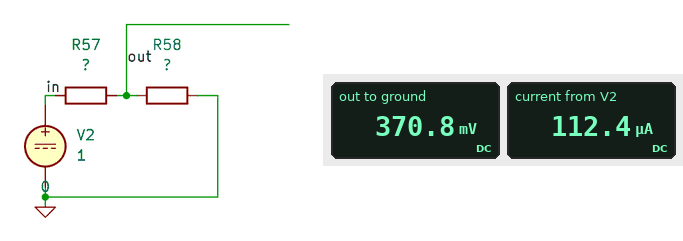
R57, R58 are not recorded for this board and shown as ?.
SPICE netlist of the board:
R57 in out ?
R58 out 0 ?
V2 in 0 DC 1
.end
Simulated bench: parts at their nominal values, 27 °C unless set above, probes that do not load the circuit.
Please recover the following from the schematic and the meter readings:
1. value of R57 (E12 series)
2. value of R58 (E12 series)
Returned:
5.6 kΩ
3.3 kΩ
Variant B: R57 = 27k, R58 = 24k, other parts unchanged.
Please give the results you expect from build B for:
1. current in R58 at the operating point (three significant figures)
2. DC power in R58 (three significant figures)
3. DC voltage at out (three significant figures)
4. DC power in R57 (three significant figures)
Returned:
19.6 µA
9.23 µW
471 mV
10.4 µW
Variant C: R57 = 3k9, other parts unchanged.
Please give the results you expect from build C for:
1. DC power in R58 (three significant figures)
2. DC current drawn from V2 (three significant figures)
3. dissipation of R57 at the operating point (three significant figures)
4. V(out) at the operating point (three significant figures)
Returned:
63.7 µW
139 µA
75.2 µW
458 mV
